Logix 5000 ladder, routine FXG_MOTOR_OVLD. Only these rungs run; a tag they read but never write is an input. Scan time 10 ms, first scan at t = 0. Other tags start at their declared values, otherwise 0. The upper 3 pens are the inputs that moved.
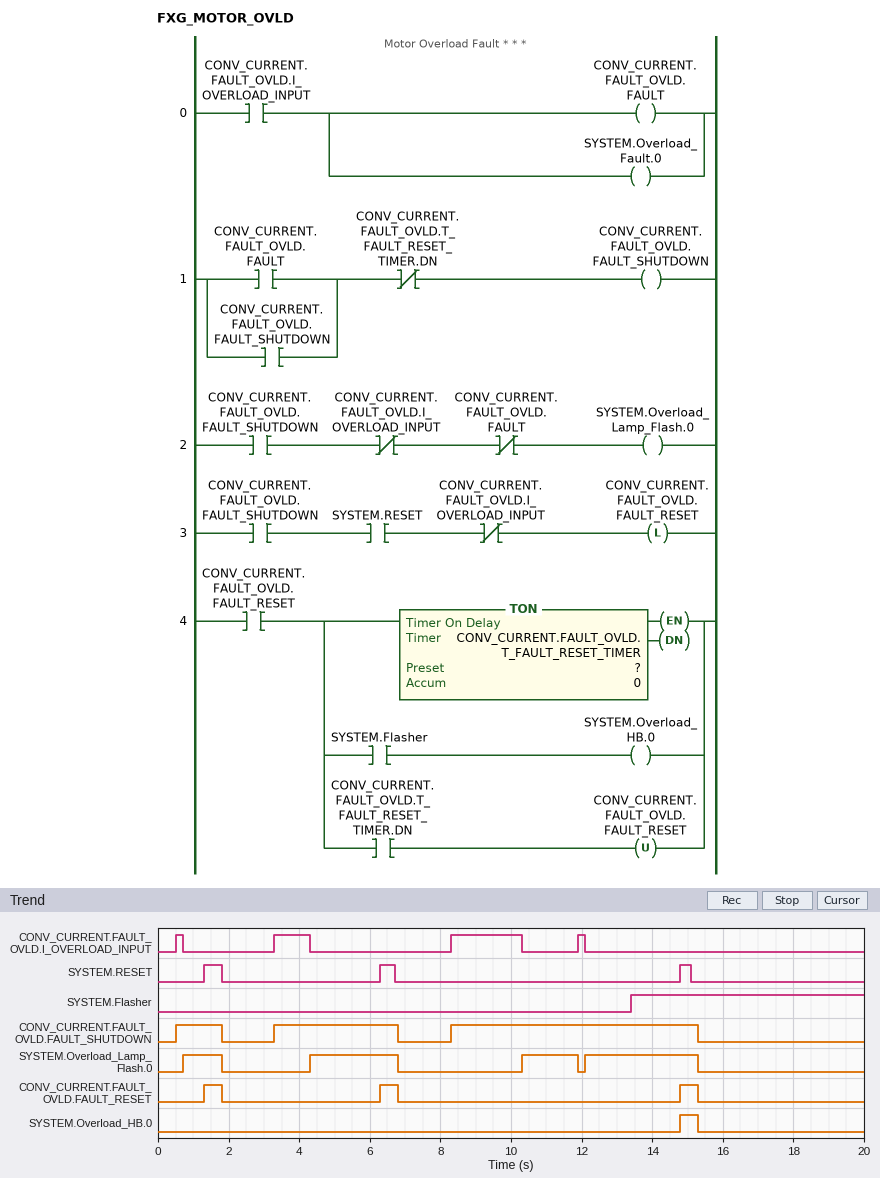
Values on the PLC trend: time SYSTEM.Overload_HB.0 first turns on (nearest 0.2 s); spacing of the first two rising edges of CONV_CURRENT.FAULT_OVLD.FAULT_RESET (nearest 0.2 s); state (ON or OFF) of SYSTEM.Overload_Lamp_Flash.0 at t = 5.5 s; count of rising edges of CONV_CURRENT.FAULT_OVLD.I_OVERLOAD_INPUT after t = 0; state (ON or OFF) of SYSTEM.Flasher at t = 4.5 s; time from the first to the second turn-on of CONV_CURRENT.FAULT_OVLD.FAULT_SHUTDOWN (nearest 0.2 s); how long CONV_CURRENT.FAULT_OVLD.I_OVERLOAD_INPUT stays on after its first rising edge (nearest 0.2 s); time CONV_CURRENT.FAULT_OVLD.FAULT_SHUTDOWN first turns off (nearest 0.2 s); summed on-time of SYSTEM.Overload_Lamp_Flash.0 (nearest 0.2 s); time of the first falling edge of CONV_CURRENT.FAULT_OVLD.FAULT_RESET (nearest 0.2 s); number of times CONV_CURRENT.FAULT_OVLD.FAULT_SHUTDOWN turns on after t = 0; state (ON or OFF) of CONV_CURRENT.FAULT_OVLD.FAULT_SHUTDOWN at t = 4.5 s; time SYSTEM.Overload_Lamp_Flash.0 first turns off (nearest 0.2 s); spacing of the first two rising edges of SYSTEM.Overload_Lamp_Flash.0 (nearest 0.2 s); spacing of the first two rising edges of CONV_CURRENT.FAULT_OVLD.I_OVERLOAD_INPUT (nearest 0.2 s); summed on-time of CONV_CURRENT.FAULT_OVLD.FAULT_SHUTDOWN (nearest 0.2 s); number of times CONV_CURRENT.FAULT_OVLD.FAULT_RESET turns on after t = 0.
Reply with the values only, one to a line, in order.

14.8 s
5.0 s
ON
4
OFF
2.8 s
0.2 s
1.8 s
8.4 s
1.8 s
3
ON
1.8 s
3.6 s
2.8 s
11.8 s
3
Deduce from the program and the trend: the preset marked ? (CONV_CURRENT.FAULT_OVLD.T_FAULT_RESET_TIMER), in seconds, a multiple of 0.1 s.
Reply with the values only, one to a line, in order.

0.5 s
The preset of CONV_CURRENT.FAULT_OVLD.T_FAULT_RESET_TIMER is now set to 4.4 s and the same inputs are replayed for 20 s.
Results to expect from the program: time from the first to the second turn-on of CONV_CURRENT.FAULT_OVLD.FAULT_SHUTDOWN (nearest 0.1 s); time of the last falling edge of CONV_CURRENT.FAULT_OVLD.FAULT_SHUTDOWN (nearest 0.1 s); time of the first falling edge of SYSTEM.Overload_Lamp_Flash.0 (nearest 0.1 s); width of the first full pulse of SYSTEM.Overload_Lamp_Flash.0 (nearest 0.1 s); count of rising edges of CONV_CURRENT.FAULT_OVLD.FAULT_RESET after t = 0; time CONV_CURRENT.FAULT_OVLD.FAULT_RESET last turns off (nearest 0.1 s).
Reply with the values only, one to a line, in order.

7.8 s
19.2 s
3.3 s
2.6 s
2
19.2 s
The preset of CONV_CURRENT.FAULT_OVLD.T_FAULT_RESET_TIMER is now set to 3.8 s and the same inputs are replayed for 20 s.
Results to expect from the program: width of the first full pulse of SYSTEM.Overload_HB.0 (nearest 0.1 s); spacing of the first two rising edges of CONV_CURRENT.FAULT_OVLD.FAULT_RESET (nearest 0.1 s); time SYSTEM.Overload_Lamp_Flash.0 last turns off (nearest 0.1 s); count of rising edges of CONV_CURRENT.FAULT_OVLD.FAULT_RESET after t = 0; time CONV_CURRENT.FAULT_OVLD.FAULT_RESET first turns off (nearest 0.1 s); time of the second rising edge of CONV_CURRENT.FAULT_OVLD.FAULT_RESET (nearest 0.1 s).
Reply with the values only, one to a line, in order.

3.8 s
13.5 s
18.6 s
2
5.1 s
14.8 s
